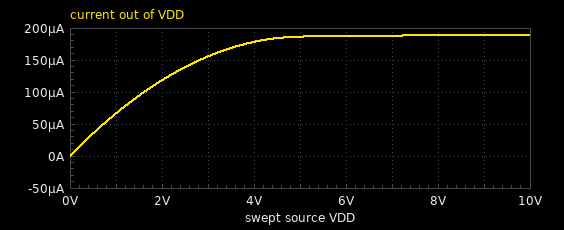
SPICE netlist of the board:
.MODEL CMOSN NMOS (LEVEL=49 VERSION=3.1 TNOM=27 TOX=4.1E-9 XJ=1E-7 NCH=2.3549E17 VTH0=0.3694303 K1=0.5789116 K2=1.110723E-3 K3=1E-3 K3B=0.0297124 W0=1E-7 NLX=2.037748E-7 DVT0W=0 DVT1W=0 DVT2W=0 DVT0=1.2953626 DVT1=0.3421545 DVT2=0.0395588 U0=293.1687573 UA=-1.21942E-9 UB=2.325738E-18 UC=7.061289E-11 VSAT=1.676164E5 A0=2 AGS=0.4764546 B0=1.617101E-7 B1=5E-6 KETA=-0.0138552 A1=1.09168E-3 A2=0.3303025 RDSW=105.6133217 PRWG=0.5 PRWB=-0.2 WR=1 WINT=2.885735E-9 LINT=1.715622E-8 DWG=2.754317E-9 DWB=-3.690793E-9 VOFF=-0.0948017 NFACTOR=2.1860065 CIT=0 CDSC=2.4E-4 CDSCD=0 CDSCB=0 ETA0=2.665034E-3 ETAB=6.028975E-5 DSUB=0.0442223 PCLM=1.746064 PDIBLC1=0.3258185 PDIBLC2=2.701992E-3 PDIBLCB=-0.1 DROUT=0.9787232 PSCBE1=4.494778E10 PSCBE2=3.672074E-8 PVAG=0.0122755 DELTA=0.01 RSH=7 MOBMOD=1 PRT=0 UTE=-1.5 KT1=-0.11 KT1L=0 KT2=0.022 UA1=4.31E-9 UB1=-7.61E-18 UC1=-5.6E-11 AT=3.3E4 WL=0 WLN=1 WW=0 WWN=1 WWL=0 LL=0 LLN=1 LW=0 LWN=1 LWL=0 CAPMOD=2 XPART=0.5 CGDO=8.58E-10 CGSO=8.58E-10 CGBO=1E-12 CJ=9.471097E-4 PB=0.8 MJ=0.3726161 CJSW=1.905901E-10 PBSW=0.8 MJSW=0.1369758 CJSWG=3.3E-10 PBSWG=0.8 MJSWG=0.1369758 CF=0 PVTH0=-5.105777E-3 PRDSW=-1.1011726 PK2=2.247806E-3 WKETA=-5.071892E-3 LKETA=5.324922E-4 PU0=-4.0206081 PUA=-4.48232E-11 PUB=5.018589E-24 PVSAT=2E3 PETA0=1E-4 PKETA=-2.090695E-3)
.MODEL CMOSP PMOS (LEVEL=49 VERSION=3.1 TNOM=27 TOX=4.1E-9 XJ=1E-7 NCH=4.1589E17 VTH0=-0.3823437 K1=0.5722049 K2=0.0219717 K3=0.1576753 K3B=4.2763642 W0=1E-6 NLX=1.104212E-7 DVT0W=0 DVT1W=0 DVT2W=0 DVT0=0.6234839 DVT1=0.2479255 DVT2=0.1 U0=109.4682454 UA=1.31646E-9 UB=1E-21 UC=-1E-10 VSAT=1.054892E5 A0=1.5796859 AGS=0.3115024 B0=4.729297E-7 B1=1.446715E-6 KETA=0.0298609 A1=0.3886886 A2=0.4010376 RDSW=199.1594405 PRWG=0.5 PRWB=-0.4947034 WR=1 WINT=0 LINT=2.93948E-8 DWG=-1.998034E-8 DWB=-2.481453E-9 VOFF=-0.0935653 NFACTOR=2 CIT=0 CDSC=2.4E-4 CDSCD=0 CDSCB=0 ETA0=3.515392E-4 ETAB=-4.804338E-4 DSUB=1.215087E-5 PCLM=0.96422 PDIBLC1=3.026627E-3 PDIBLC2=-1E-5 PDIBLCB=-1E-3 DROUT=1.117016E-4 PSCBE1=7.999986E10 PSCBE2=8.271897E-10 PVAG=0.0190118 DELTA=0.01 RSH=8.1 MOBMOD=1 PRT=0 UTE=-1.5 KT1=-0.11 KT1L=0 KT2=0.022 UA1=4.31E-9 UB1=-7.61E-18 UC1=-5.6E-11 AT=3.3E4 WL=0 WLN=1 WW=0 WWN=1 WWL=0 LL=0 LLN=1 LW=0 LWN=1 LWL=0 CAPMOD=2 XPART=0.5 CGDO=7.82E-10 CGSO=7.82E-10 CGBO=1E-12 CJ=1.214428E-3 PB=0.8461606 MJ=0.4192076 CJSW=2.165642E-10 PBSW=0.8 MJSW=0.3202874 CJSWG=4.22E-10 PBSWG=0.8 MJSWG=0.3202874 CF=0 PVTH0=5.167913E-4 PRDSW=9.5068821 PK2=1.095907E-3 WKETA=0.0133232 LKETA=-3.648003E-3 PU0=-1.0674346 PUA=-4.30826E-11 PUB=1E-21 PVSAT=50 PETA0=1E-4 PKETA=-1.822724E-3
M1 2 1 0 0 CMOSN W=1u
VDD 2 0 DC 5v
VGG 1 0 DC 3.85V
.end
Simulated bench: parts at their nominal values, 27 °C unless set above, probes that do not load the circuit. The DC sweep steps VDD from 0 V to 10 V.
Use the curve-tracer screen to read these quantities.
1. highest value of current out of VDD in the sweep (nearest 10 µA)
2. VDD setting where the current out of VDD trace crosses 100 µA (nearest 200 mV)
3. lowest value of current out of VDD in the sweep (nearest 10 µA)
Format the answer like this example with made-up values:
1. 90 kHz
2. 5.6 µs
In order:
1. 190 µA
2. 1.6 V
3. 0 A
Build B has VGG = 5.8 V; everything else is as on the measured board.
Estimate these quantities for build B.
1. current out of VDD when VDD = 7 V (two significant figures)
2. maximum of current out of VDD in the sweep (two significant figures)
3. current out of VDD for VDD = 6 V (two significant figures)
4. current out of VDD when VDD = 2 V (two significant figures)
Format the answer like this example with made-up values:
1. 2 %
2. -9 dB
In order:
1. 350 µA
2. 470 µA
3. 310 µA
4. 110 µA
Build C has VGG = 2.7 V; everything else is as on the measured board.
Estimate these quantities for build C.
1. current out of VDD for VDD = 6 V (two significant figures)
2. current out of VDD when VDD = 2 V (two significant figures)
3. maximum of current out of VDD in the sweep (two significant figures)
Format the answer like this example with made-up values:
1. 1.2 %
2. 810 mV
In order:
1. 95 µA
2. 91 µA
3. 96 µA
